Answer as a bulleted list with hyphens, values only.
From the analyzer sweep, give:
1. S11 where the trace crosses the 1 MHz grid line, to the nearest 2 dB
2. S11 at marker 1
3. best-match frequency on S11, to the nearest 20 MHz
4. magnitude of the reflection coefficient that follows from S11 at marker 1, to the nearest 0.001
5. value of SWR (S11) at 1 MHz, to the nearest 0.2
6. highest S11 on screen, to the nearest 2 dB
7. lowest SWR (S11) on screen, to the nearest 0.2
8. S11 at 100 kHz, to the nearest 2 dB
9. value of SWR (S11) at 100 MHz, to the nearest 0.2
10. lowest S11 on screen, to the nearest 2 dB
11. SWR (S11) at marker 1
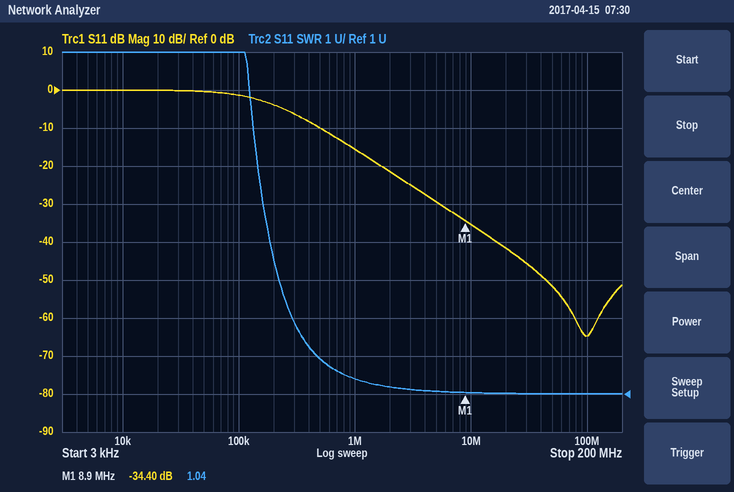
- -16 dB
- -34.40 dB
- 100 MHz
- 0.019
- 1.4
- 0 dB
- 1.0
- -2 dB
- 1.0
- -64 dB
- 1.04
